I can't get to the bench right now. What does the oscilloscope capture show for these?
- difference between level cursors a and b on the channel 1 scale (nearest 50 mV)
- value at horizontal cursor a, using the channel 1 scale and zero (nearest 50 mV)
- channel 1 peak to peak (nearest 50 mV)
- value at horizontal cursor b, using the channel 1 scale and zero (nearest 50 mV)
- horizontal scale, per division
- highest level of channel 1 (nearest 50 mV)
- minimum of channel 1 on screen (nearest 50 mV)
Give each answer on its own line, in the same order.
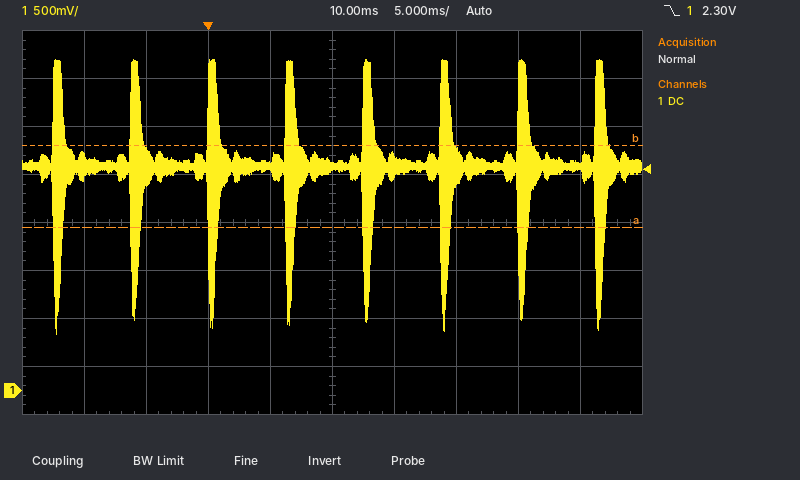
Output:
850 mV
1.70 V
2.85 V
2.55 V
5 ms
3.45 V
600 mV
